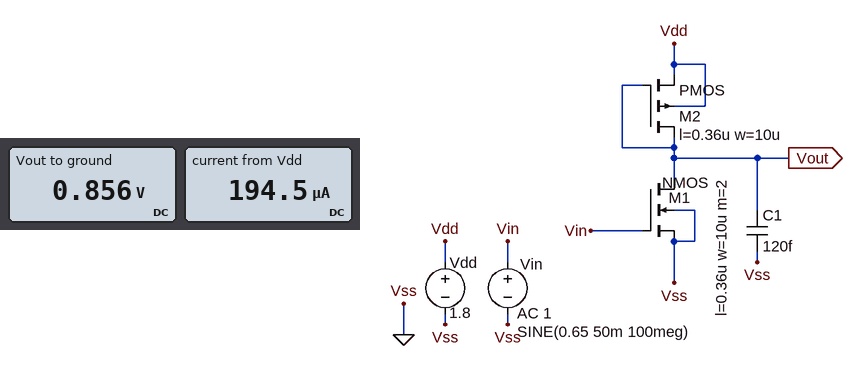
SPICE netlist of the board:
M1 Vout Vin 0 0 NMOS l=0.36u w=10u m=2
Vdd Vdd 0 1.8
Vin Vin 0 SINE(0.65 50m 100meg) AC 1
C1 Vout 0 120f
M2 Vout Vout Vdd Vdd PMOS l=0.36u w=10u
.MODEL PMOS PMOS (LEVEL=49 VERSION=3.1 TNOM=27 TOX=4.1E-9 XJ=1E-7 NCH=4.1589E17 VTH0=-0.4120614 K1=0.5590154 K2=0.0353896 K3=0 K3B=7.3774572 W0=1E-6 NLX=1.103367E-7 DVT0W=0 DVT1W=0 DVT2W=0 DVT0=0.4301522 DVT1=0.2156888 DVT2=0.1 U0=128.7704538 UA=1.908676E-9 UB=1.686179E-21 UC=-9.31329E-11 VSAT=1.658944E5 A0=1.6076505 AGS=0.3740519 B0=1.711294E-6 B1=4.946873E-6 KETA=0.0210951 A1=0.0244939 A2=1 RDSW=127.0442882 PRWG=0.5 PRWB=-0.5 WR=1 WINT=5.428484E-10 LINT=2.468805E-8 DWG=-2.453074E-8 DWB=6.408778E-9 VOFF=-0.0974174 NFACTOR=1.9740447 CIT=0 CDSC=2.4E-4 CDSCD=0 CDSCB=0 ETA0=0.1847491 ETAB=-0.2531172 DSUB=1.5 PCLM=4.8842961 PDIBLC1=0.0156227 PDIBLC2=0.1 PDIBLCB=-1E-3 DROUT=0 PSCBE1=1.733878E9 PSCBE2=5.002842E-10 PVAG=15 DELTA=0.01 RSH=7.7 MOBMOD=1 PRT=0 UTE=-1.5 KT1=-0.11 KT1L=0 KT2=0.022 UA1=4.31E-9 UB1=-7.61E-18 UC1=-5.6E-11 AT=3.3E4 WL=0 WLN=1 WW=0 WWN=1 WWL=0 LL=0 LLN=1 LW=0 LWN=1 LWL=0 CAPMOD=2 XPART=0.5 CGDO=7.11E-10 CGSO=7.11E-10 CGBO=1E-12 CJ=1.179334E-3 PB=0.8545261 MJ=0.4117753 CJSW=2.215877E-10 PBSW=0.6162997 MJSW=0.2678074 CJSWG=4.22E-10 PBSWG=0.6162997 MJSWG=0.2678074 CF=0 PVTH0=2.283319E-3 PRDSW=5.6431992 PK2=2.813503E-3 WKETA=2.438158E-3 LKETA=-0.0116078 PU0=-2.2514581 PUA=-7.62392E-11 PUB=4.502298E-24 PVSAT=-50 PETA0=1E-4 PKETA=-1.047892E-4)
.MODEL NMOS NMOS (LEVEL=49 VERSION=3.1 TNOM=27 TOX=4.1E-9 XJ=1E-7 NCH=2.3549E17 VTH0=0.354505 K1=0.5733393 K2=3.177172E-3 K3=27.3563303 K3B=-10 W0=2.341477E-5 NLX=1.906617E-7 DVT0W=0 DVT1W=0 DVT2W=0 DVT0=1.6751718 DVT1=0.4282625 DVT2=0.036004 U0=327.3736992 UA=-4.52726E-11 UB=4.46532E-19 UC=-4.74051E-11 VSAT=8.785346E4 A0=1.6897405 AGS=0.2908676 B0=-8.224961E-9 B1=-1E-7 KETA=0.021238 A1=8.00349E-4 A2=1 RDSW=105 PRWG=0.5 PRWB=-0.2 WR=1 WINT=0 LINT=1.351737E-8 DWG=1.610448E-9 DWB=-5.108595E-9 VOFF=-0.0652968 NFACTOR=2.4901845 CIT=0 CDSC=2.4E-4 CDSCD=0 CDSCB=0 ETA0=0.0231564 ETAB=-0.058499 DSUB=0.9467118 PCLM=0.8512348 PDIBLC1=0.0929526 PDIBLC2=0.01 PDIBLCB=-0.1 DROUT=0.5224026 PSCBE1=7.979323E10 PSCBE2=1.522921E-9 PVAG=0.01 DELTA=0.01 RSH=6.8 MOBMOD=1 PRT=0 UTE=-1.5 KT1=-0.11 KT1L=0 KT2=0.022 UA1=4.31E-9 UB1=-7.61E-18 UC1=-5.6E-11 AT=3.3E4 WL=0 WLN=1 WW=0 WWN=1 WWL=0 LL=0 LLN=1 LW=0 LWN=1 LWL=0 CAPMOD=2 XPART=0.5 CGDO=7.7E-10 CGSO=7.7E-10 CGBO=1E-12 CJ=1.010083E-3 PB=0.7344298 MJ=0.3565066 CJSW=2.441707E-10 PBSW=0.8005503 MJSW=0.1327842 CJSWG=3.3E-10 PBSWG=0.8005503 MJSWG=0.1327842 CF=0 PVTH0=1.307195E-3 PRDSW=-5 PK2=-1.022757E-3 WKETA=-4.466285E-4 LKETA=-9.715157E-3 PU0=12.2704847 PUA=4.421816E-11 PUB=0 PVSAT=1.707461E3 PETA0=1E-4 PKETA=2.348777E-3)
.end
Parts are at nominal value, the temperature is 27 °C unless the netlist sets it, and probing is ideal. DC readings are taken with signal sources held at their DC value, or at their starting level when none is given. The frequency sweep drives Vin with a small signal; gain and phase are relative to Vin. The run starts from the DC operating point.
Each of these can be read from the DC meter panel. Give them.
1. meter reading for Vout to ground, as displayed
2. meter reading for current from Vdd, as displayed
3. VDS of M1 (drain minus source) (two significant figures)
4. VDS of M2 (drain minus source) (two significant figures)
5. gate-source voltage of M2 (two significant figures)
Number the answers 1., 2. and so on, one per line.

1. 0.856 V
2. 194.5 µA
3. 860 mV
4. -940 mV
5. -940 mV
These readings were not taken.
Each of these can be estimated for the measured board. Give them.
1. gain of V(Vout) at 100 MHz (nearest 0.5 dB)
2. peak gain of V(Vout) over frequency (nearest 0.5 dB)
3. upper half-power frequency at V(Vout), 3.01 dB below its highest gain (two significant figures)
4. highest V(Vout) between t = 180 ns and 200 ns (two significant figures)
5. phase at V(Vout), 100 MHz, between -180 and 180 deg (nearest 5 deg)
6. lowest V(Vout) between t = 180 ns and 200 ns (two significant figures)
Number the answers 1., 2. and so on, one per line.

1. 10.0 dB
2. 10.0 dB
3. 730 MHz
4. 1.0 V
5. 170 deg
6. 700 mV
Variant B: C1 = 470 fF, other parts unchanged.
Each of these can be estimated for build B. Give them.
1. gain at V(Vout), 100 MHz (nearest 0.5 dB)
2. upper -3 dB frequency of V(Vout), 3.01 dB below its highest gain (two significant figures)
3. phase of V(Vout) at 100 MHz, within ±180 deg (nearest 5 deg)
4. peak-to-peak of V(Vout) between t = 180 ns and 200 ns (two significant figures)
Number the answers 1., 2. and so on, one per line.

1. 9.0 dB
2. 230 MHz
3. 155 deg
4. 280 mV
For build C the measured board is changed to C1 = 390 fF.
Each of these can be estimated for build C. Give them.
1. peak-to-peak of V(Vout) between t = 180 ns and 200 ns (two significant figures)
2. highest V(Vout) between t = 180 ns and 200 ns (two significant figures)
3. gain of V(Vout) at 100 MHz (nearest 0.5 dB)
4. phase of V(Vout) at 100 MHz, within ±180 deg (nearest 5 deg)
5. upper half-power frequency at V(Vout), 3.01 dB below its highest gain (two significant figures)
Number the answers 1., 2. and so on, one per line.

1. 290 mV
2. 990 mV
3. 9.5 dB
4. 160 deg
5. 280 MHz
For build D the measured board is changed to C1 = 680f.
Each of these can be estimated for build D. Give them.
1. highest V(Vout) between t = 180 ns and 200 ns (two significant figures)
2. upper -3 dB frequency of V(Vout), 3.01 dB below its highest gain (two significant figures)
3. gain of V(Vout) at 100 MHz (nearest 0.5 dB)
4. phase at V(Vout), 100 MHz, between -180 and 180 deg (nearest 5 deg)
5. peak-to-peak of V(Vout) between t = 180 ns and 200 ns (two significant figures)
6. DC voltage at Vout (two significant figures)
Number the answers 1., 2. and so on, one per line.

1. 980 mV
2. 170 MHz
3. 8.5 dB
4. 150 deg
5. 260 mV
6. 860 mV
